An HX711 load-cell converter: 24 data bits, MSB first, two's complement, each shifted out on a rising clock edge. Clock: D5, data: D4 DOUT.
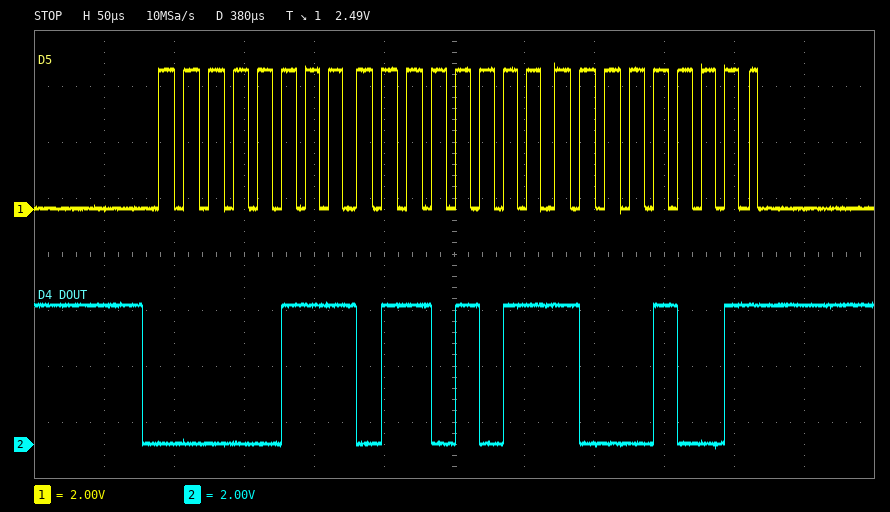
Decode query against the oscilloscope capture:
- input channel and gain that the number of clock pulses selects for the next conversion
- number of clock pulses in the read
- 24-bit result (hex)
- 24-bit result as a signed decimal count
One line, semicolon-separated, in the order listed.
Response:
channel A, gain 128; 25; 0x076B89; 486281
